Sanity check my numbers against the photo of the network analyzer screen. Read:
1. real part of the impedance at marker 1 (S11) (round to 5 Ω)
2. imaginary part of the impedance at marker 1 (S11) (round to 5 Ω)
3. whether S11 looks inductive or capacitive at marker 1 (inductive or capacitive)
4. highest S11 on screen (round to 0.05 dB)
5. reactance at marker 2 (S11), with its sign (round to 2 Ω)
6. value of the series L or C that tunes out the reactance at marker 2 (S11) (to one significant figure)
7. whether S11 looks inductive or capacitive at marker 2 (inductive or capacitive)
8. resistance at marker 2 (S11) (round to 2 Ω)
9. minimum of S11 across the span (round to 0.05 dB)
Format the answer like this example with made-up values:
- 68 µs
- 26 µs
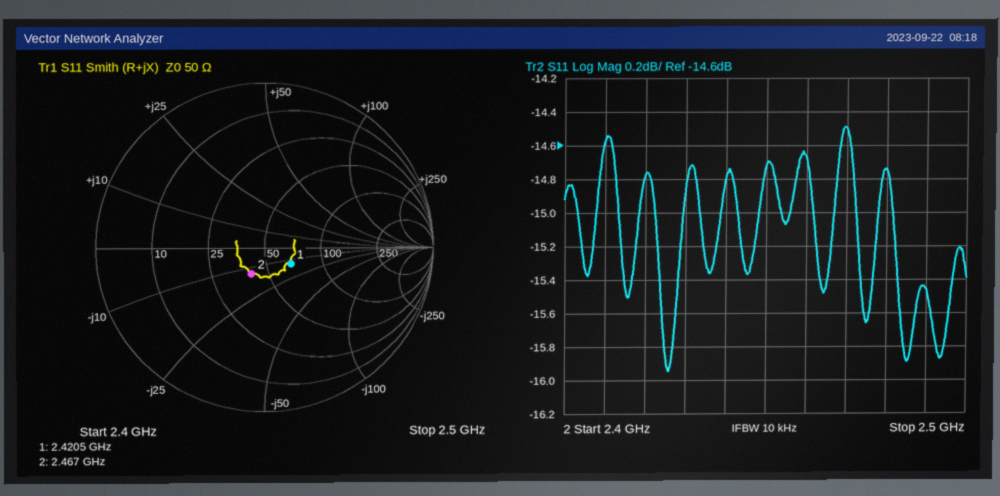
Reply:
- 65 Ω
- -15 Ω
- capacitive
- -14.50 dB
- -14 Ω
- 900 pH
- capacitive
- 40 Ω
- -15.95 dB
